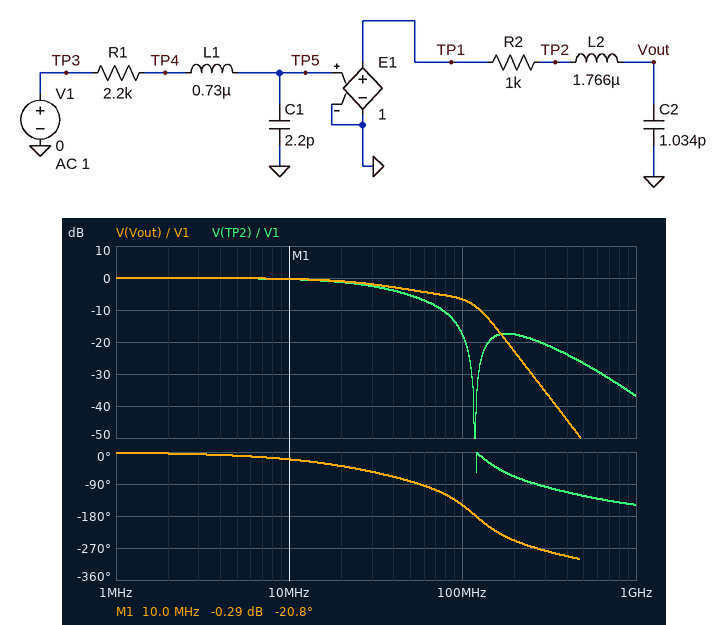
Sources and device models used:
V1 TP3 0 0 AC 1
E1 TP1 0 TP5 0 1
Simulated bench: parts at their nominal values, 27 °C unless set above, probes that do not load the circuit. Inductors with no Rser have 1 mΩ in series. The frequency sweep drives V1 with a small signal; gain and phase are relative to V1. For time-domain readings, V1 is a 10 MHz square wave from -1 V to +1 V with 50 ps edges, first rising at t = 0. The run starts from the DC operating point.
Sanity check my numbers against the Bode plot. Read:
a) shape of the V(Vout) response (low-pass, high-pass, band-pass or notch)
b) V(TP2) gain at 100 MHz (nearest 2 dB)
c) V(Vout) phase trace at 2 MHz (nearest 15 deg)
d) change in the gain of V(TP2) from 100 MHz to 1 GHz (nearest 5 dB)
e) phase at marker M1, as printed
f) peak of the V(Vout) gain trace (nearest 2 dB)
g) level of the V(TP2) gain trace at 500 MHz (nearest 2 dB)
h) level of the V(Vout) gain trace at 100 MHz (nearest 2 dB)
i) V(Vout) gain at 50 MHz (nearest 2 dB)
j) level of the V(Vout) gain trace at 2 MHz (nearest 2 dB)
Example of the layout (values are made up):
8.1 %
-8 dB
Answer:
low-pass
-18 dB
0 deg
-20 dB
-20.8 deg
0 dB
-26 dB
-6 dB
-4 dB
0 dB
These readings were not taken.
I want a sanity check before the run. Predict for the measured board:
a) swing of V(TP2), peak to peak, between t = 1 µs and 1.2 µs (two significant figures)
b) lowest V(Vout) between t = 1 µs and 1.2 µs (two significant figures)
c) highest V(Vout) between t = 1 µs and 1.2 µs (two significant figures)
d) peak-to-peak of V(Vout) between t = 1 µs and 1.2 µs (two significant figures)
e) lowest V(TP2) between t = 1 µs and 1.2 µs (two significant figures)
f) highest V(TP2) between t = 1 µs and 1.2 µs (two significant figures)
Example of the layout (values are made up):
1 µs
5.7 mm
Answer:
2.0 V
-1.0 V
1.0 V
2.0 V
-1.0 V
1.0 V
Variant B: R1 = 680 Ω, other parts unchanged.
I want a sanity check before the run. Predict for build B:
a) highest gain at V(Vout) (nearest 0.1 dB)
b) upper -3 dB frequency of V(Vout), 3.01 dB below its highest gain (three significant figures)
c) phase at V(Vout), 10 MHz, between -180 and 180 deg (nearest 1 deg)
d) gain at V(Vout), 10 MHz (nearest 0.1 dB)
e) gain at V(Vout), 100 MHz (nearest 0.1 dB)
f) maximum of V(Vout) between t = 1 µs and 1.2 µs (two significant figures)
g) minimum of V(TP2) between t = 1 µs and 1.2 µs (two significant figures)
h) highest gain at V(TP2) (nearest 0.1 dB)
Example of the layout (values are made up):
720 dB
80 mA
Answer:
3.1 dB
126 MHz
-9 deg
0.1 dB
2.9 dB
1.6 V
-1.3 V
0 dB
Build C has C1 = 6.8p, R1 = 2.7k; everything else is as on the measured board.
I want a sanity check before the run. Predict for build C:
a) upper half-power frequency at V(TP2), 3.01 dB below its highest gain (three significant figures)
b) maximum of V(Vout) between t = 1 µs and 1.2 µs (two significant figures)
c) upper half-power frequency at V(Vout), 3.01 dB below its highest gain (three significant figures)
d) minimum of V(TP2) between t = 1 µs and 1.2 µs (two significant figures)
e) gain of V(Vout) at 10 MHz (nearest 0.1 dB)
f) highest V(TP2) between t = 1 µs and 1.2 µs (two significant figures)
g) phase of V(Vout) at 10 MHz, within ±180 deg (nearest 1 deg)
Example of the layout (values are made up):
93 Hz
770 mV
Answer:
8.77 MHz
880 mV
8.87 MHz
-870 mV
-3.6 dB
870 mV
-53 deg
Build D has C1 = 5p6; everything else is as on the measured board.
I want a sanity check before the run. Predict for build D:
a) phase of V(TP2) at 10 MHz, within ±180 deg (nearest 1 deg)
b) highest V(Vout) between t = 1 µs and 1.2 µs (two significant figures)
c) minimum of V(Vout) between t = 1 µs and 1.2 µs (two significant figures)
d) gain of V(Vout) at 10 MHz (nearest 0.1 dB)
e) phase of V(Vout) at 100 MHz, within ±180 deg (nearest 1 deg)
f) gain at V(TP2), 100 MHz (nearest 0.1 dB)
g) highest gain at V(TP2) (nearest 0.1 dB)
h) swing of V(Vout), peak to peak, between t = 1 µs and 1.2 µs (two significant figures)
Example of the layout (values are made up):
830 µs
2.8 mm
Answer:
-42 deg
970 mV
-970 mV
-1.9 dB
-161 deg
-25.9 dB
0 dB
1.9 V
